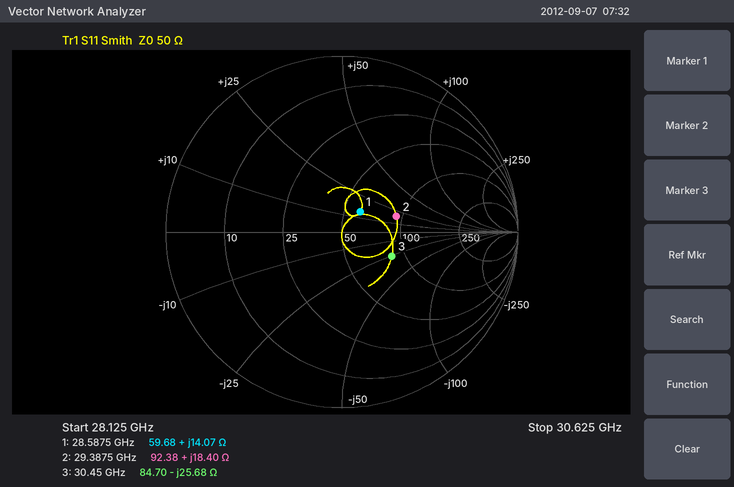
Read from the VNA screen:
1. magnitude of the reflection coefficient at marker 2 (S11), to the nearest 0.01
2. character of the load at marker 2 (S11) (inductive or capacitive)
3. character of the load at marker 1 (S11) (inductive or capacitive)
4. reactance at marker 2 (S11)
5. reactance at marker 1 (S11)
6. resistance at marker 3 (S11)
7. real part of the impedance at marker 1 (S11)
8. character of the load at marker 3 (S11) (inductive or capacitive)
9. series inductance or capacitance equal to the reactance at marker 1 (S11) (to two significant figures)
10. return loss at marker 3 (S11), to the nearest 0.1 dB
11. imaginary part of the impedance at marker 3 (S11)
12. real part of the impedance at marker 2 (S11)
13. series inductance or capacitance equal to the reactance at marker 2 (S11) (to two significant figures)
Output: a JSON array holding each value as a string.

["0.32", "inductive", "inductive", "+18.40 Ω", "+14.07 Ω", "84.70 Ω", "59.68 Ω", "capacitive", "78 pH", "10.0 dB", "-25.68 Ω", "92.38 Ω", "100 pH"]
